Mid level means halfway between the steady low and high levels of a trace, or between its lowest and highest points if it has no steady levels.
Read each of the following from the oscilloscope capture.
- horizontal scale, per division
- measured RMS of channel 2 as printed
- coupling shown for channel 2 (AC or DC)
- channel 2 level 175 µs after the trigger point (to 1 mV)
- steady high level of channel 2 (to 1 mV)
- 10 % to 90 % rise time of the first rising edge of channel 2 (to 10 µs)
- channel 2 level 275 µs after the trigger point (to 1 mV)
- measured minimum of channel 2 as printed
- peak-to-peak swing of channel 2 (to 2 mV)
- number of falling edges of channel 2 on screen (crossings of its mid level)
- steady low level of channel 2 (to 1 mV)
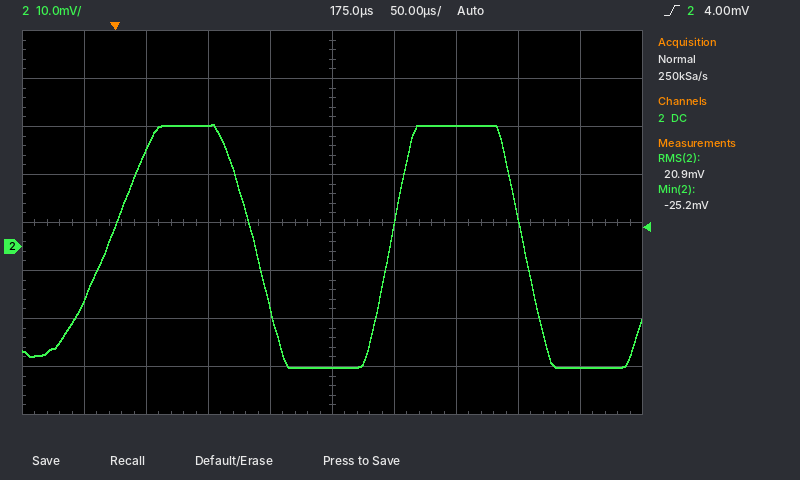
50 µs
20.9 mV
DC
-25 mV
25 mV
70 µs
25 mV
-25.2 mV
50 mV
2
-25 mV
